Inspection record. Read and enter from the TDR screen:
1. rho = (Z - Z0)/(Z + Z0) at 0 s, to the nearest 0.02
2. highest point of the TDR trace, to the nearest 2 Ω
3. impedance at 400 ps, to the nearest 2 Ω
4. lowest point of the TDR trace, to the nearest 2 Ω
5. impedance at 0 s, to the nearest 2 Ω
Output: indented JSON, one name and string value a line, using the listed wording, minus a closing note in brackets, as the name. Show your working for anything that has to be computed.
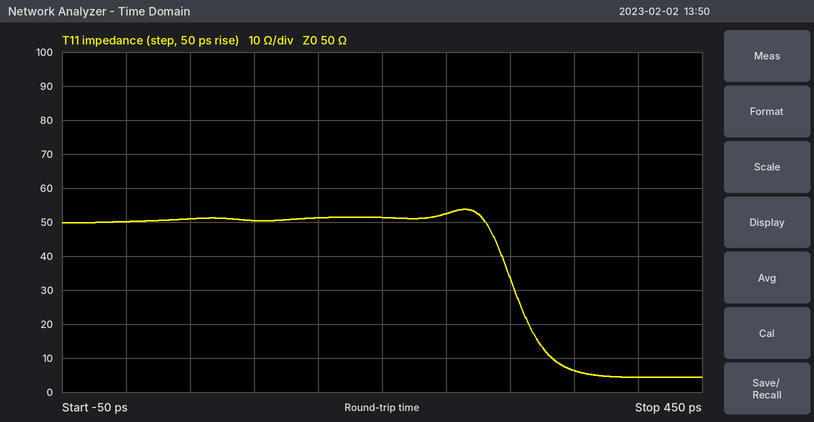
{
  "rho = (Z - Z0)/(Z + Z0) at 0 s, to the nearest 0.02": "(50 − 50)/(50 + 50) ≈ 0.00",
  "highest point of the TDR trace, to the nearest 2 Ω": "54 Ω",
  "impedance at 400 ps, to the nearest 2 Ω": "4 Ω",
  "lowest point of the TDR trace, to the nearest 2 Ω": "4 Ω",
  "impedance at 0 s, to the nearest 2 Ω": "50 Ω"
}
